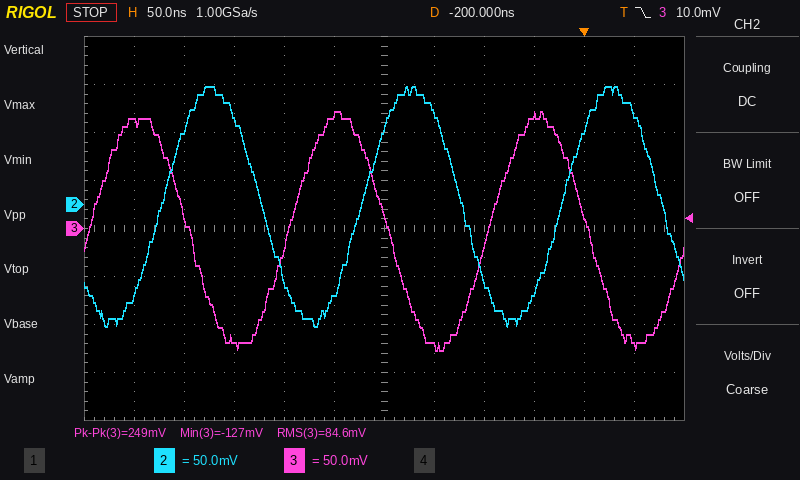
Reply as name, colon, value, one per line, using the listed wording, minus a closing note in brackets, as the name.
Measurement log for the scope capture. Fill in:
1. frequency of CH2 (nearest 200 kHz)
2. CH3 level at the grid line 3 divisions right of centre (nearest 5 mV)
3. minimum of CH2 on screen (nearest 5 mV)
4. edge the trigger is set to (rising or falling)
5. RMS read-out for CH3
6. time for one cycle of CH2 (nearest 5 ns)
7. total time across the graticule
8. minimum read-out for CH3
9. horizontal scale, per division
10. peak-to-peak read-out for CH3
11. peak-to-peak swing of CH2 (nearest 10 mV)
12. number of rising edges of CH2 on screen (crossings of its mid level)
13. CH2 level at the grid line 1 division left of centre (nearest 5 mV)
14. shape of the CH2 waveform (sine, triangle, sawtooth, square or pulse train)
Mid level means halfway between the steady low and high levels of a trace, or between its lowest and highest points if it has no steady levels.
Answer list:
frequency of CH2: 5.0 MHz
CH3 level at the grid line 3 divisions right of centre: 120 mV
minimum of CH2 on screen: -125 mV
edge the trigger is set to: falling
RMS read-out for CH3: 84.6 mV
time for one cycle of CH2: 200 ns
total time across the graticule: 600 ns
minimum read-out for CH3: -127 mV
horizontal scale, per division: 50 ns
peak-to-peak read-out for CH3: 249 mV
peak-to-peak swing of CH2: 250 mV
number of rising edges of CH2 on screen: 3
CH2 level at the grid line 1 division left of centre: -95 mV
shape of the CH2 waveform: sine
